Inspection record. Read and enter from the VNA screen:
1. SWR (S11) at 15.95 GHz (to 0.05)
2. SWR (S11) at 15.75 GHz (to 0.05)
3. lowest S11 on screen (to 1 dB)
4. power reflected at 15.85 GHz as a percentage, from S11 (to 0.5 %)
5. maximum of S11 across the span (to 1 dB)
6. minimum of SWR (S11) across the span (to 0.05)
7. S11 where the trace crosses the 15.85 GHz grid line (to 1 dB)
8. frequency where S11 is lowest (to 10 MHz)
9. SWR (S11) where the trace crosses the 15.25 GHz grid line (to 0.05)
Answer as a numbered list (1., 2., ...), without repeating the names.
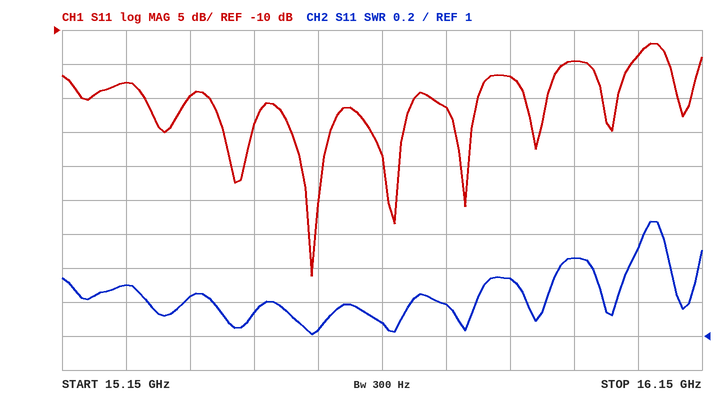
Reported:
1. 1.45
2. 1.20
3. -46 dB
4. 2.0 %
5. -12 dB
6. 1.00
7. -17 dB
8. 15.54 GHz
9. 1.30
